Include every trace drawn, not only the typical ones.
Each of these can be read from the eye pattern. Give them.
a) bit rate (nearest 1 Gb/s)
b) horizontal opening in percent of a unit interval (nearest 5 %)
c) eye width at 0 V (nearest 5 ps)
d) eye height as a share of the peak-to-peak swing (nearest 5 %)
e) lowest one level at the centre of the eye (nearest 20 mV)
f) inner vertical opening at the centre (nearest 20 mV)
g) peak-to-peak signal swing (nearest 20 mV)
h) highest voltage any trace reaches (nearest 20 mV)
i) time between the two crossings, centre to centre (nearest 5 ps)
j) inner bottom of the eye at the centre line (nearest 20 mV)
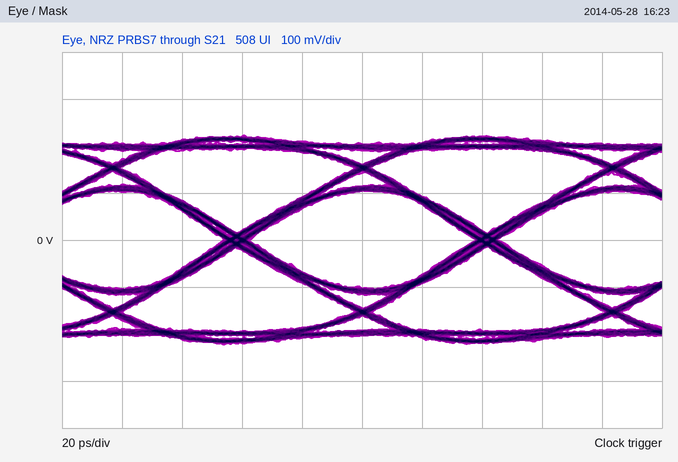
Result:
12 Gb/s
90 %
75 ps
45 %
100 mV
200 mV
440 mV
220 mV
85 ps
-100 mV
